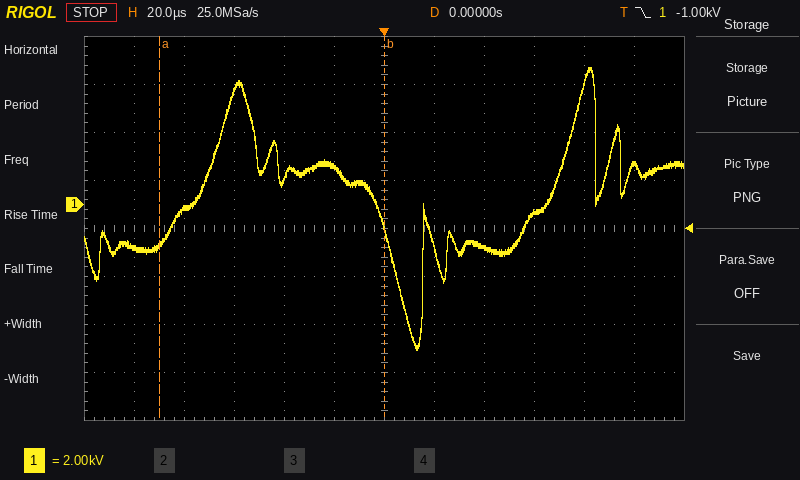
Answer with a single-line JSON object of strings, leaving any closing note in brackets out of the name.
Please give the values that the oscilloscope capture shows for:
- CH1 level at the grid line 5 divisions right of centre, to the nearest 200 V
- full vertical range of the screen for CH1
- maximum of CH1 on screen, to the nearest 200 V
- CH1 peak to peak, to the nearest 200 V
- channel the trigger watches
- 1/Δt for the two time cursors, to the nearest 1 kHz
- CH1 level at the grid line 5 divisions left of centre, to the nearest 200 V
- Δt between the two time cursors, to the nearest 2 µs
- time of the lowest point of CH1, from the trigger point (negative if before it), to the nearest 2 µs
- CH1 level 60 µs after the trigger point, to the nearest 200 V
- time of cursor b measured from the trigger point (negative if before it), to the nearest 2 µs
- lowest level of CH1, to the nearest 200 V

{"CH1 level at the grid line 5 divisions right of centre, to the nearest 200 V": "1.6 kV", "full vertical range of the screen for CH1": "16 kV", "maximum of CH1 on screen, to the nearest 200 V": "5.8 kV", "CH1 peak to peak, to the nearest 200 V": "11.8 kV", "channel the trigger watches": "CH1", "1/Δt for the two time cursors, to the nearest 1 kHz": "11 kHz", "CH1 level at the grid line 5 divisions left of centre, to the nearest 200 V": "-1.8 kV", "Δt between the two time cursors, to the nearest 2 µs": "90 µs", "time of the lowest point of CH1, from the trigger point (negative if before it), to the nearest 2 µs": "+14 µs", "CH1 level 60 µs after the trigger point, to the nearest 200 V": "-400 V", "time of cursor b measured from the trigger point (negative if before it), to the nearest 2 µs": "0 µs", "lowest level of CH1, to the nearest 200 V": "-6.0 kV"}
